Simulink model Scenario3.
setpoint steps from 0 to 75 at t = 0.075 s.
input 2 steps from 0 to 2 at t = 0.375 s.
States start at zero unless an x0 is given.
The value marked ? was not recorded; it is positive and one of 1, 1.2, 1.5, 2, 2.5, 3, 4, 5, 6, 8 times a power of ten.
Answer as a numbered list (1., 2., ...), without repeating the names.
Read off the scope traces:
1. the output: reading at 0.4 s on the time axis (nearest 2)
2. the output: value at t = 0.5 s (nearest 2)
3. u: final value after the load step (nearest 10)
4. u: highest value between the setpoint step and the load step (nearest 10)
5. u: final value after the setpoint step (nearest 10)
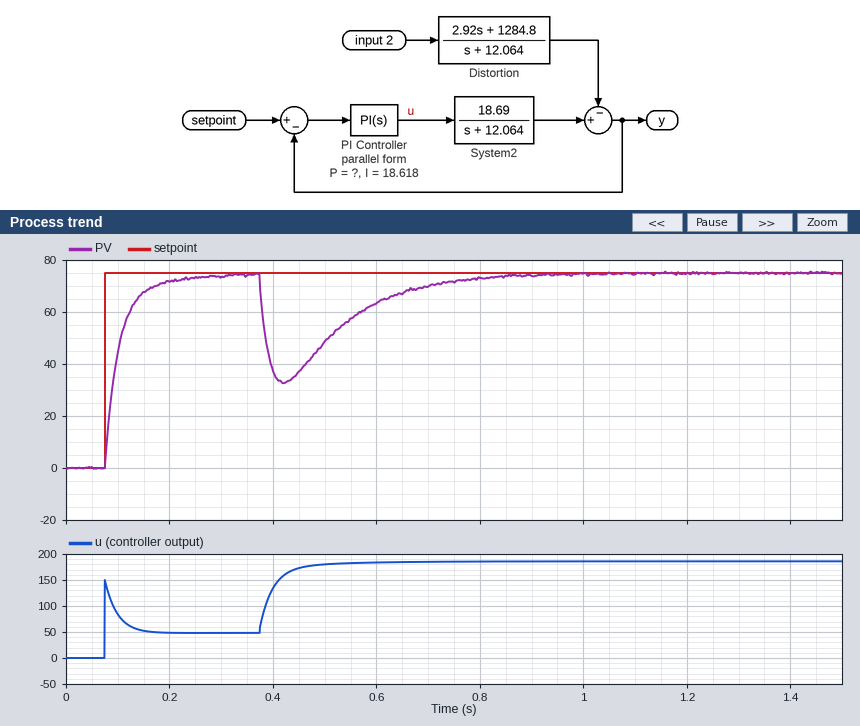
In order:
1. 38
2. 48
3. 190
4. 150
5. 50
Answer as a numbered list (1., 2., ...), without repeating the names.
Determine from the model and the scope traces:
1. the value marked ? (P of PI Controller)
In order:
1. 2
